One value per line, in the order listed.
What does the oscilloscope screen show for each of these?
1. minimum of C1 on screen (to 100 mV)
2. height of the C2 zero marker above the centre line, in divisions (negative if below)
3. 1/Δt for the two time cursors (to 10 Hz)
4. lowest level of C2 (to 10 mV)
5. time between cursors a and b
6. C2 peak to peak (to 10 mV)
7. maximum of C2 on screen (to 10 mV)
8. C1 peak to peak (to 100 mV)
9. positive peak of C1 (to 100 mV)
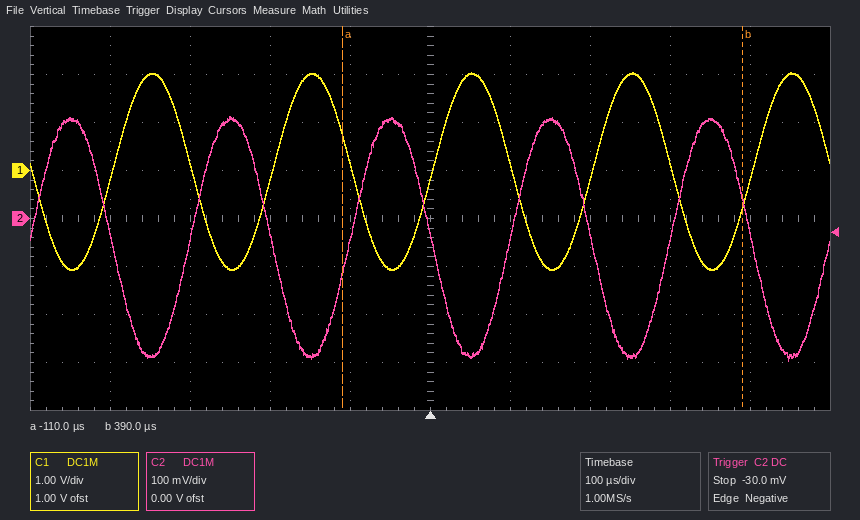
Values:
-2.1 V
0.0 div
2.00 kHz
-300 mV
500 µs
510 mV
210 mV
4.1 V
2.0 V
